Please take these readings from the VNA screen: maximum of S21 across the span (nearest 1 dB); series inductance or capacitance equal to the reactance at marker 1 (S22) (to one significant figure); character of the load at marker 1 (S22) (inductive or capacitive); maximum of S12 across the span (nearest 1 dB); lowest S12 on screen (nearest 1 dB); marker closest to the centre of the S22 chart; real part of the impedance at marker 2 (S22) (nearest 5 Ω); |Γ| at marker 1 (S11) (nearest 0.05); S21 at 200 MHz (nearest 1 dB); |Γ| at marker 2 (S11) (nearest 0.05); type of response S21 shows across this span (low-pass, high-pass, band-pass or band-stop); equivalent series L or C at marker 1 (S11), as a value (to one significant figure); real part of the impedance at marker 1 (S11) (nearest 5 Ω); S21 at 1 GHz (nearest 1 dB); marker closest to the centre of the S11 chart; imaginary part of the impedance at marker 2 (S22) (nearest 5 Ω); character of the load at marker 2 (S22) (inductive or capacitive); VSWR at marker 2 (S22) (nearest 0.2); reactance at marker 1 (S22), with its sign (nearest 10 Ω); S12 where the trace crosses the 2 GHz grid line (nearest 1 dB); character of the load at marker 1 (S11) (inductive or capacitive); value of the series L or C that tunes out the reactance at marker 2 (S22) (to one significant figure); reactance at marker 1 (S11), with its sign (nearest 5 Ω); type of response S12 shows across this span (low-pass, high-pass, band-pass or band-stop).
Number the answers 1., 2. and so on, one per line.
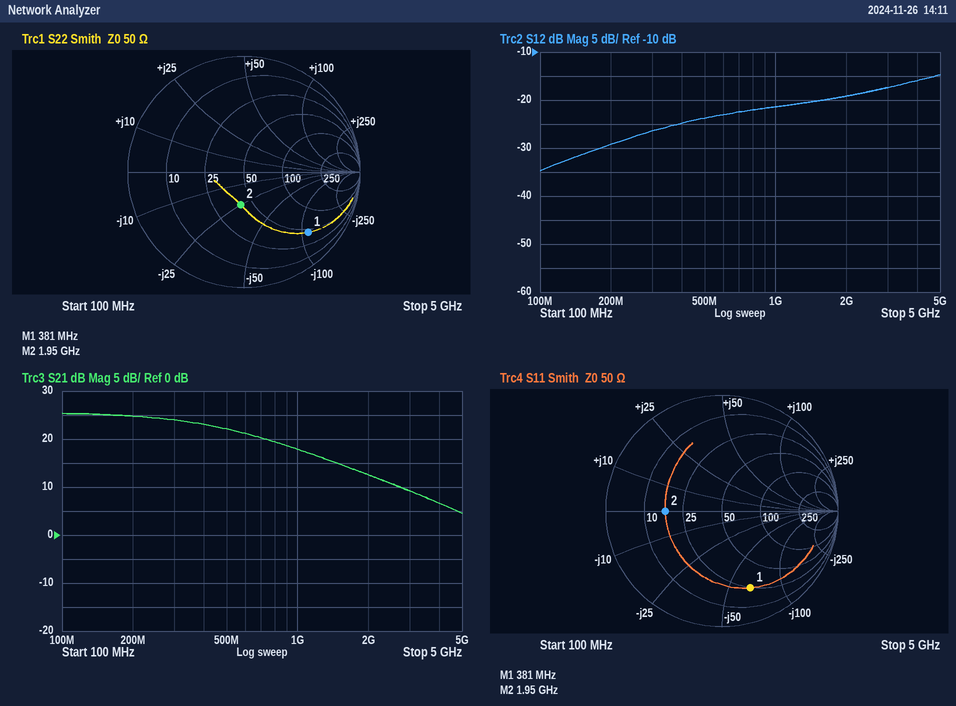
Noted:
1. 25 dB
2. 4 pF
3. capacitive
4. -15 dB
5. -35 dB
6. marker 2
7. 40 Ω
8. 0.70
9. 25 dB
10. 0.50
11. low-pass
12. 6 pF
13. 25 Ω
14. 18 dB
15. marker 2
16. -25 Ω
17. capacitive
18. 1.8
19. -110 Ω
20. -19 dB
21. capacitive
22. 2 nH
23. -65 Ω
24. high-pass
